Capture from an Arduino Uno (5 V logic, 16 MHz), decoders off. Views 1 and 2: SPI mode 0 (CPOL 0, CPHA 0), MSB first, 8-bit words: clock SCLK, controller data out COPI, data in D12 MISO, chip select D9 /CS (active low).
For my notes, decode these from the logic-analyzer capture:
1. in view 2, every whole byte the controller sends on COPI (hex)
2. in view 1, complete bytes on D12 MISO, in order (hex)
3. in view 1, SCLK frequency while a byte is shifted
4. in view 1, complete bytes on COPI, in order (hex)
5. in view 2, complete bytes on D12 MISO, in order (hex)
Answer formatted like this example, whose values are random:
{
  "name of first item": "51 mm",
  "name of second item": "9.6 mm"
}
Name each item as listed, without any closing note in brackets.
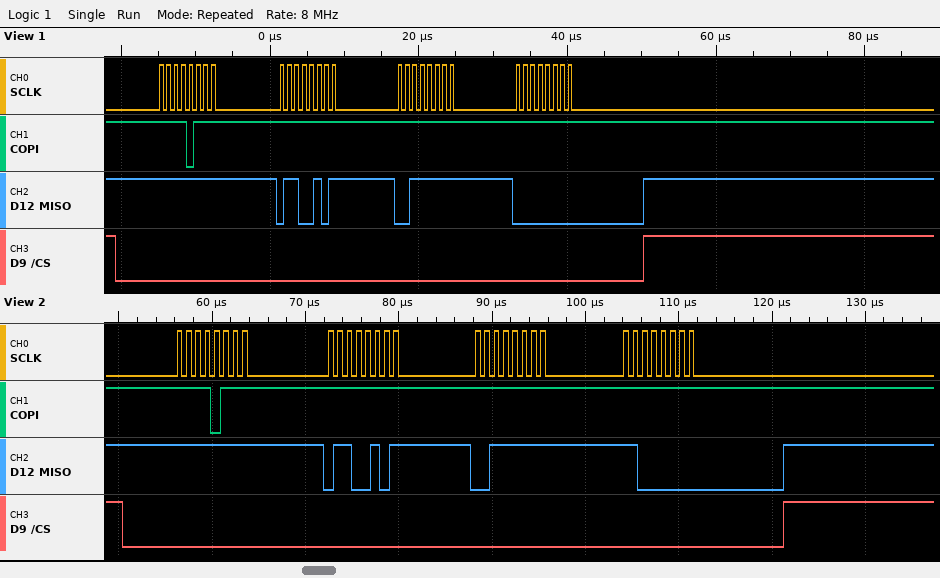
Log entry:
{
  "in view 2, every whole byte the controller sends on COPI": "F7 FF FF FF",
  "in view 1, complete bytes on D12 MISO, in order": "FF 65 3F 00",
  "in view 1, SCLK frequency while a byte is shifted": "1 MHz",
  "in view 1, complete bytes on COPI, in order": "F7 FF FF FF",
  "in view 2, complete bytes on D12 MISO, in order": "FF 65 3F C0"
}
